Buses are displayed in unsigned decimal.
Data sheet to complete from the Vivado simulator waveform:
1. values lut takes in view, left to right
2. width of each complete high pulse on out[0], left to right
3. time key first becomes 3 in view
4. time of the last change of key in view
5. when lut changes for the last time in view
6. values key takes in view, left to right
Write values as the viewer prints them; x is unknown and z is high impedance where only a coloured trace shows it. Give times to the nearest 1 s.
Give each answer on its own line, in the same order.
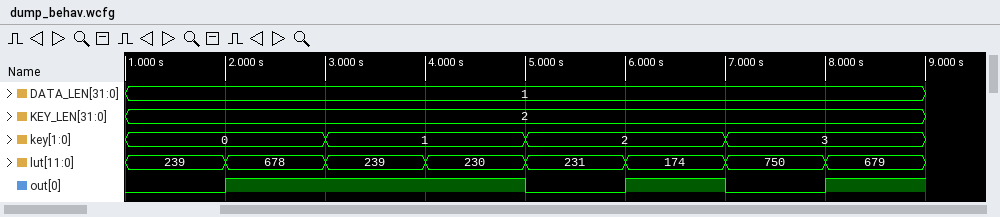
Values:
239, 678, 239, 230, 231, 174, 750, 679
3 s, 1 s
7 s
7 s
8 s
0, 1, 2, 3
